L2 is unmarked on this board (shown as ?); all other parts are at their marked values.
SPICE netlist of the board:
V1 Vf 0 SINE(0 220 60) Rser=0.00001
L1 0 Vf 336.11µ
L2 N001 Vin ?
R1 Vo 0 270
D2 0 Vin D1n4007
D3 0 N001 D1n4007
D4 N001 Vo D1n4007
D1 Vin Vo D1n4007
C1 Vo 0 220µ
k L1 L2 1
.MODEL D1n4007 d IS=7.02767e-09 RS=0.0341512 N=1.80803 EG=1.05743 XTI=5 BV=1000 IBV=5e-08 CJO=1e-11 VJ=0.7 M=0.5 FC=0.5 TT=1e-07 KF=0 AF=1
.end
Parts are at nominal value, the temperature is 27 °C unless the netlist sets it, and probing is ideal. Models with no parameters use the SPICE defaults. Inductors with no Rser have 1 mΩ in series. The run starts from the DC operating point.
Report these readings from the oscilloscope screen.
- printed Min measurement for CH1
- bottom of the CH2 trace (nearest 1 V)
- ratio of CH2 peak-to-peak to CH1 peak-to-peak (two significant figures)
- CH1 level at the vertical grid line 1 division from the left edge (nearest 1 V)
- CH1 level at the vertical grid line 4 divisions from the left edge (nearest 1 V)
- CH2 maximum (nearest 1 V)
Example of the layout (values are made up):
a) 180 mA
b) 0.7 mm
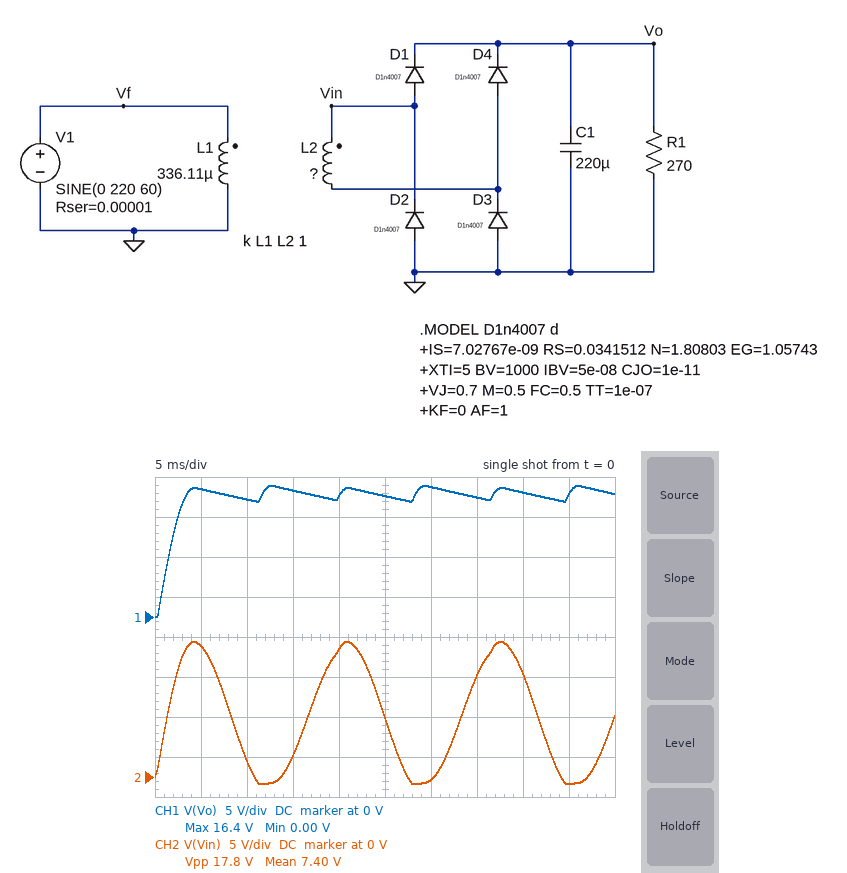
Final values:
a) 0.00 V
b) -1 V
c) 1.1
d) 16 V
e) 15 V
f) 17 V
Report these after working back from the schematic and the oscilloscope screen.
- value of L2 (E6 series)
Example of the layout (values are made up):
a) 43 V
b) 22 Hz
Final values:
a) 2.2 µH
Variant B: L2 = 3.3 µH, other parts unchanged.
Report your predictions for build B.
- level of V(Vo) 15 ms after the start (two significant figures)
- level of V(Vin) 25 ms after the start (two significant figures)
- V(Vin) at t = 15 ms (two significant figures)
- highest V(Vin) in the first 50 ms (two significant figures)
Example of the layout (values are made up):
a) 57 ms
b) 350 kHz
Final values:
a) 20 V
b) 9.2 V
c) 3.4 V
d) 21 V
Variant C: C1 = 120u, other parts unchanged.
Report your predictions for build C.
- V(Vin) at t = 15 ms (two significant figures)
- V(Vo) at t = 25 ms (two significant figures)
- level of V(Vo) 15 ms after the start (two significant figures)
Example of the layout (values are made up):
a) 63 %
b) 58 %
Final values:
a) 2.4 V
b) 14 V
c) 15 V
